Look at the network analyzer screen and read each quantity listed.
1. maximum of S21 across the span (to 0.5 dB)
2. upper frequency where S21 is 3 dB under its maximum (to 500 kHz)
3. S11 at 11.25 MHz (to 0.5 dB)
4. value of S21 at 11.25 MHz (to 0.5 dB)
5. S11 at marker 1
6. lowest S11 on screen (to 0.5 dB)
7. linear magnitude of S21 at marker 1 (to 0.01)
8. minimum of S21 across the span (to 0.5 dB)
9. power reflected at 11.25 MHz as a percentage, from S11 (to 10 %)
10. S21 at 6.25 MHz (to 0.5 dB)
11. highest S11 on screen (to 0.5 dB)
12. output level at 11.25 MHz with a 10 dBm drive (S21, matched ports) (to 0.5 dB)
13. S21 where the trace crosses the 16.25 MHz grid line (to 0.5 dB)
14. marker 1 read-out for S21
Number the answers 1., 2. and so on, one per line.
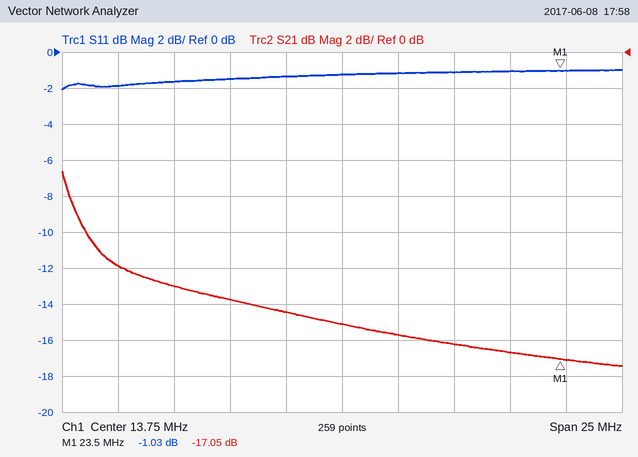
1. -6.5 dB
2. 2.0 MHz
3. -1.5 dB
4. -14.5 dB
5. -1.03 dB
6. -2.0 dB
7. 0.14
8. -17.5 dB
9. 70 %
10. -13.0 dB
11. -1.0 dB
12. -4.5 dBm
13. -15.5 dB
14. -17.05 dB
